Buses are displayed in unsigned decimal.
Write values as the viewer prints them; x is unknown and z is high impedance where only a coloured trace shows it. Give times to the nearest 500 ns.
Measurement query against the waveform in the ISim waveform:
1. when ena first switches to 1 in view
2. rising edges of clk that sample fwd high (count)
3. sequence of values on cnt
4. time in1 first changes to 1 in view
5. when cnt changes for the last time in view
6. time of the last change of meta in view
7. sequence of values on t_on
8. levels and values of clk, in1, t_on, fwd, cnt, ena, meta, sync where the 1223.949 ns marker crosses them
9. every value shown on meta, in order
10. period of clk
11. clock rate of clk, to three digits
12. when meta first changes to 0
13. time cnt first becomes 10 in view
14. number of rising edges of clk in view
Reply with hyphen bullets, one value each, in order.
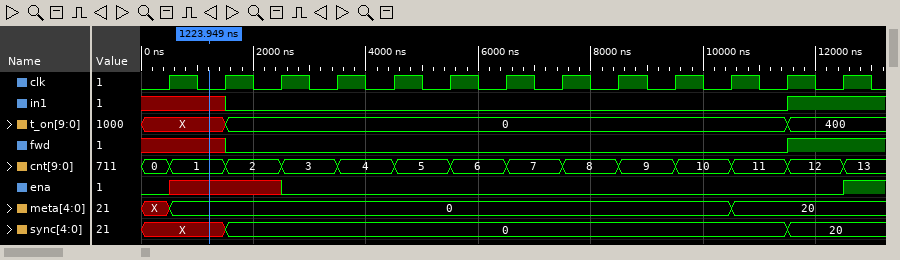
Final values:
- 12500 ns
- 1
- 0, 1, 2, 3, 4, 5, 6, 7, 8, 9, 10, 11, 12, 13
- 11500 ns
- 12500 ns
- 10500 ns
- X, 0, 400
- clk=0, in1=x, t_on=X, fwd=x, cnt=1, ena=x, meta=0, sync=X
- X, 0, 20
- 1000 ns
- 1.00 MHz
- 500 ns
- 9500 ns
- 13
